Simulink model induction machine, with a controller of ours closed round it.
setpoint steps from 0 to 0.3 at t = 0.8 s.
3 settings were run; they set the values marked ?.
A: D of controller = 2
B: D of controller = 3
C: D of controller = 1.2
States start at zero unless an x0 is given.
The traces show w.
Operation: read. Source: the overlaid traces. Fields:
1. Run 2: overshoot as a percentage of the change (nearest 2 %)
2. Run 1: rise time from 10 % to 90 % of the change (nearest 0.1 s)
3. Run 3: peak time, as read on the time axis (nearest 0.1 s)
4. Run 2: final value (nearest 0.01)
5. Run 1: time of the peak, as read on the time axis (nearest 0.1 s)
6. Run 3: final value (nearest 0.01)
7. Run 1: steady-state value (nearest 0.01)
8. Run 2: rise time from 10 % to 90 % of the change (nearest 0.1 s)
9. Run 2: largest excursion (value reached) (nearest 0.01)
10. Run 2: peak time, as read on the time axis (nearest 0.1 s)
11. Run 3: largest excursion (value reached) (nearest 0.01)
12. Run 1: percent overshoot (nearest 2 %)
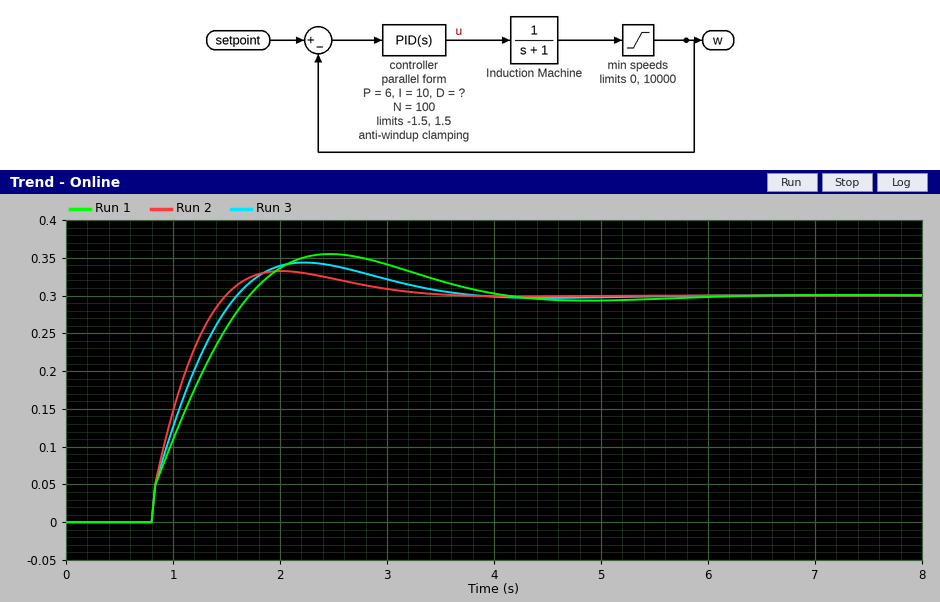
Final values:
10 %
0.7 s
2.2 s
0.30
2.5 s
0.30
0.30
0.5 s
0.33
2.0 s
0.34
18 %
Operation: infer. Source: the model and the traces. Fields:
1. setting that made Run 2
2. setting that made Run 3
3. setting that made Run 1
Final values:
C
A
B
